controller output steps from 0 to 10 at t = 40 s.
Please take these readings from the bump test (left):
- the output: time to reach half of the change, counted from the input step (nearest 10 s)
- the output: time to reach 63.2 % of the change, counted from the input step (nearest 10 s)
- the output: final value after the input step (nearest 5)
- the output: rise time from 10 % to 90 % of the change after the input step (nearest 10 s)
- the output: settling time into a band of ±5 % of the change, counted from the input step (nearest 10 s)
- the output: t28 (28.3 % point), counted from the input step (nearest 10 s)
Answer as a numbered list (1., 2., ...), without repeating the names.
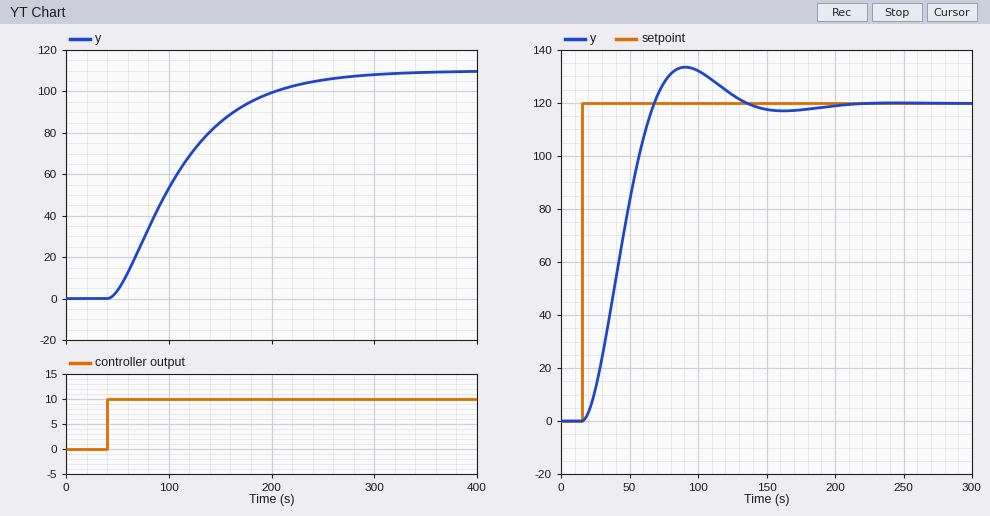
1. 60 s
2. 80 s
3. 110
4. 140 s
5. 200 s
6. 40 s
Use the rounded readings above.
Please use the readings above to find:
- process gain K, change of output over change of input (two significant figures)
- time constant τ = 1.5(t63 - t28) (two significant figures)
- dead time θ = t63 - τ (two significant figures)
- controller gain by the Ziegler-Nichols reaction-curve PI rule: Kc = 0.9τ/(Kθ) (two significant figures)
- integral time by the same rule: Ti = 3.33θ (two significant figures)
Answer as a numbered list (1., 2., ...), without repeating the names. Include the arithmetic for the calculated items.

1. (110 - 0) / 10 = 11
2. 1.5 × (80 - 40) = 60 s
3. 80 - 60 = 20 s
4. 0.9 × 60 / (11 × 20) = 0.25
5. 3.33 × 20 = 67 s
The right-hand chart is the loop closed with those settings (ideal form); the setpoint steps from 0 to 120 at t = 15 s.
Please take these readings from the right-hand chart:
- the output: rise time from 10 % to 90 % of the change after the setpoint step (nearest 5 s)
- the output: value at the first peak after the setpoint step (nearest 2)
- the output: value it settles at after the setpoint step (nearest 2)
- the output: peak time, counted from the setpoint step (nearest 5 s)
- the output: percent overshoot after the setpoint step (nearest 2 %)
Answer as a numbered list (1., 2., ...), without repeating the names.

1. 35 s
2. 134
3. 120
4. 75 s
5. 12 %
